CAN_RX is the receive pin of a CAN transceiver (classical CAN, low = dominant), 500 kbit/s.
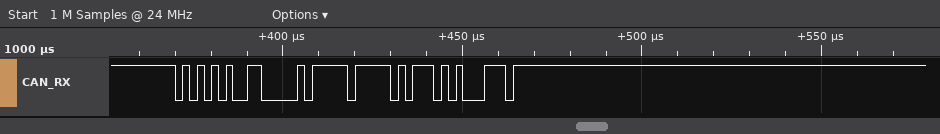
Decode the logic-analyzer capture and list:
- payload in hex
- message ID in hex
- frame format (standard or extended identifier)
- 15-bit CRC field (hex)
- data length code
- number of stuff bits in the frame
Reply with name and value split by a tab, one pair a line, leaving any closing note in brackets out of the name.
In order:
payload in hex	FF
message ID in hex	0x553
frame format	standard
15-bit CRC field	0x6EA3
data length code	1
number of stuff bits in the frame	3
